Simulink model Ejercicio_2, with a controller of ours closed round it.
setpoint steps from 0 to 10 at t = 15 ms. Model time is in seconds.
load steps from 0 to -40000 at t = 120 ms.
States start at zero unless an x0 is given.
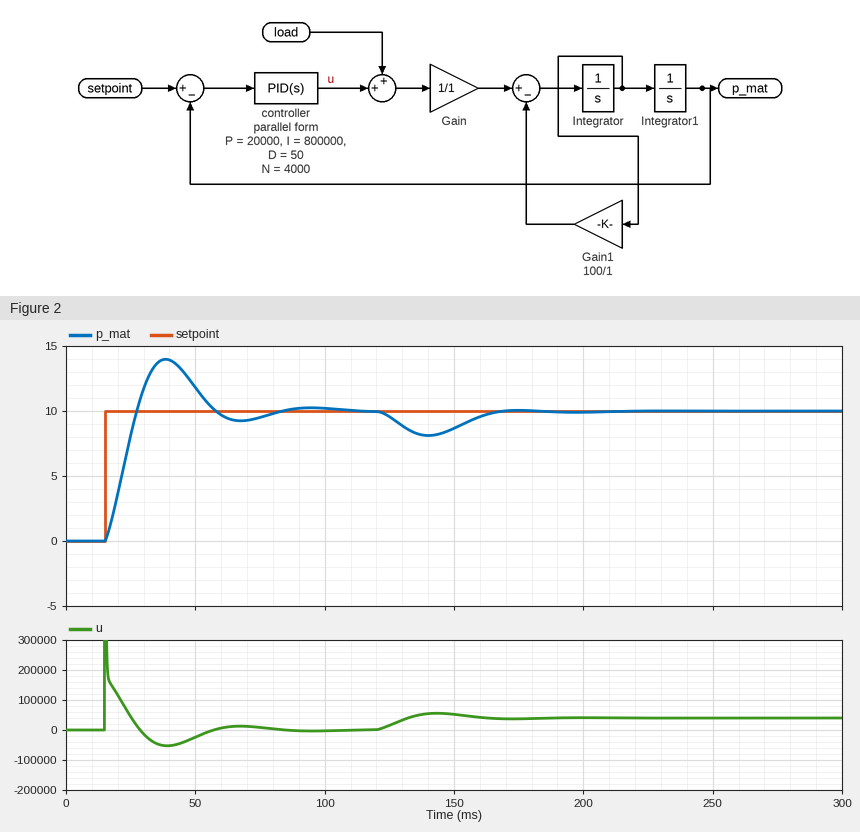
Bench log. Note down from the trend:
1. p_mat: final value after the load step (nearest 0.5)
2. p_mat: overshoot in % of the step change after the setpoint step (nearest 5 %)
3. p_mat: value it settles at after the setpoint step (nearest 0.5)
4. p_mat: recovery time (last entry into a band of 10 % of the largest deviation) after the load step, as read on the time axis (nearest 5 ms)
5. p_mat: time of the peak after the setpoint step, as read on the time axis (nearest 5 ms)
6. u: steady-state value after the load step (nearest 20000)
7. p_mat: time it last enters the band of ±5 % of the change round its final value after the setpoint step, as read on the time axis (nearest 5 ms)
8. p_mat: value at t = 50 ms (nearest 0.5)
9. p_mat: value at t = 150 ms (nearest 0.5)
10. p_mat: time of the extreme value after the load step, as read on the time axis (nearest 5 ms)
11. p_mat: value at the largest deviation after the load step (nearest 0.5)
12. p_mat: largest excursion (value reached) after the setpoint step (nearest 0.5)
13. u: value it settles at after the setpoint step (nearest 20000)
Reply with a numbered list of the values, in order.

1. 10.0
2. 40 %
3. 10.0
4. 165 ms
5. 40 ms
6. 40000
7. 75 ms
8. 12.0
9. 8.5
10. 140 ms
11. 8.0
12. 14.0
13. 0
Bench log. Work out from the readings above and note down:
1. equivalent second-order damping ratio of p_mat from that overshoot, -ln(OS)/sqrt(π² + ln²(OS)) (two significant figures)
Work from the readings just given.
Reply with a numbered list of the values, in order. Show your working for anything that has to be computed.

1. ln(0.4) = -0.916; 0.916 / sqrt(9.870 + 0.840) = 0.28
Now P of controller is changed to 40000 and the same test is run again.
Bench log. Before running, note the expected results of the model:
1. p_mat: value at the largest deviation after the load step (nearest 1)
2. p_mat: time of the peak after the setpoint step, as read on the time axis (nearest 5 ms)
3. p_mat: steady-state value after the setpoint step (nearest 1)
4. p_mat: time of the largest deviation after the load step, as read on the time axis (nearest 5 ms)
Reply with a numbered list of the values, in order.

1. 9
2. 30 ms
3. 10
4. 135 ms
